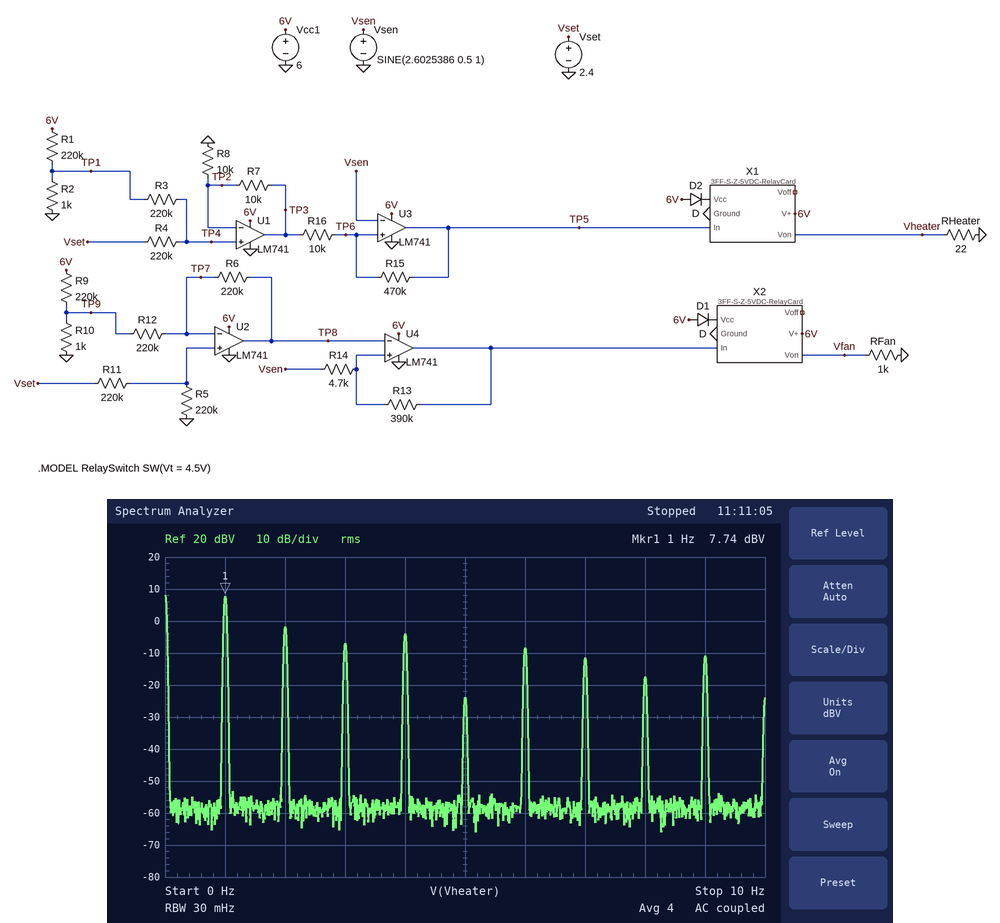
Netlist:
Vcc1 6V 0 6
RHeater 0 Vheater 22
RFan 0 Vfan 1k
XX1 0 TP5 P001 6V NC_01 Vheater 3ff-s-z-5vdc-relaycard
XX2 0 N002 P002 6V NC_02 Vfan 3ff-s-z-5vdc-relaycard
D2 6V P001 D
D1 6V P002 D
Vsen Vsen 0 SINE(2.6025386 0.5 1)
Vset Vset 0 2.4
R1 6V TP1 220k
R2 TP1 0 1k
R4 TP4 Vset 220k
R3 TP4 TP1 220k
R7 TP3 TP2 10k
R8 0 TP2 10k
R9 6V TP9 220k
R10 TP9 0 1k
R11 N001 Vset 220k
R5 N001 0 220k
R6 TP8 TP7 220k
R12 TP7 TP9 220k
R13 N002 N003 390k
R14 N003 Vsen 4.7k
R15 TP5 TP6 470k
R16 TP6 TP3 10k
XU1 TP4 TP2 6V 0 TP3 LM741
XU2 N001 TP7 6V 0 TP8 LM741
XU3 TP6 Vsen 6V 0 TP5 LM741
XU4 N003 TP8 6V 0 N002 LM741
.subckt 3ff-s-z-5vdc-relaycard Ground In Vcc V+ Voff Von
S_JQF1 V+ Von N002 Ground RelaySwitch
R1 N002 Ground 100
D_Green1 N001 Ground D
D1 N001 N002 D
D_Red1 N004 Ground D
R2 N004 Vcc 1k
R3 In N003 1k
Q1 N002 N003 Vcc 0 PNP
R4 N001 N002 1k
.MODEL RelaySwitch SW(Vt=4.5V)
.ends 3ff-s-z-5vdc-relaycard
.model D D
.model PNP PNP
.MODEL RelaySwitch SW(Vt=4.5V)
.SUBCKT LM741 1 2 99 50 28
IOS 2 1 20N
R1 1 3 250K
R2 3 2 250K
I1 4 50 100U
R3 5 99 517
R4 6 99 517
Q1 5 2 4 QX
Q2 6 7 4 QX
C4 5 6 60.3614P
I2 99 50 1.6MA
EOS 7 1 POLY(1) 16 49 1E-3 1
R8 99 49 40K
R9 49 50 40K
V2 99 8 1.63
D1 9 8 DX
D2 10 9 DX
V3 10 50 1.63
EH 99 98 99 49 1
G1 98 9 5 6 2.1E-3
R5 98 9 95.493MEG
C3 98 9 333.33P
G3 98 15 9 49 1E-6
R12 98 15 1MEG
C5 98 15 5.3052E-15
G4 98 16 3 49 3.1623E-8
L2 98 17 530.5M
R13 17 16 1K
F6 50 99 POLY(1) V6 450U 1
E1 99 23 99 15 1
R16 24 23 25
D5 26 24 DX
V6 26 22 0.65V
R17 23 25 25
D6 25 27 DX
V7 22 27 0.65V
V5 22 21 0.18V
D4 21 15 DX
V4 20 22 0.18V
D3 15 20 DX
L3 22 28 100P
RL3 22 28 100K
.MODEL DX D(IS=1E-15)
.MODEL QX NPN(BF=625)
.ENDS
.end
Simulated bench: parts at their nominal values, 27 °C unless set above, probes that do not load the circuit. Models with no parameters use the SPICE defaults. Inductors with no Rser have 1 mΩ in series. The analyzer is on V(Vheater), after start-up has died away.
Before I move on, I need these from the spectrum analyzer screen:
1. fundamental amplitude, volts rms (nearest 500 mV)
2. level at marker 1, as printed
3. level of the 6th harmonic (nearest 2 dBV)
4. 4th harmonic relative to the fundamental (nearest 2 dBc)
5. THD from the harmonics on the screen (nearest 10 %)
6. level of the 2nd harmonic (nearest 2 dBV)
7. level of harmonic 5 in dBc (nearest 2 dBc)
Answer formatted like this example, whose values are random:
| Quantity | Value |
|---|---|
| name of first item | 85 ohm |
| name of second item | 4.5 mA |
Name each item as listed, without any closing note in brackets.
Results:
| Quantity | Value |
|---|---|
| fundamental amplitude, volts rms | 2.5 V |
| level at marker 1, as printed | 7.74 dBV |
| level of the 6th harmonic | -8 dBV |
| 4th harmonic relative to the fundamental | -12 dBc |
| THD from the harmonics on the screen | 50 % |
| level of the 2nd harmonic | -2 dBV |
| level of harmonic 5 in dBc | -32 dBc |
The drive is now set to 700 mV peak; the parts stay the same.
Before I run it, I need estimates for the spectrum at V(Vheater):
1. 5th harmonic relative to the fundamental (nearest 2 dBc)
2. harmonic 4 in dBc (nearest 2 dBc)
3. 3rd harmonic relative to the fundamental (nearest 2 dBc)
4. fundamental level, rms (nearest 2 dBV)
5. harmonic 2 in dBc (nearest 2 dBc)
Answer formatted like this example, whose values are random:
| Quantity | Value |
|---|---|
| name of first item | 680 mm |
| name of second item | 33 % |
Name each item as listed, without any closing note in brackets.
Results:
| Quantity | Value |
|---|---|
| 5th harmonic relative to the fundamental | -22 dBc |
| harmonic 4 in dBc | -14 dBc |
| 3rd harmonic relative to the fundamental | -12 dBc |
| fundamental level, rms | 8 dBV |
| harmonic 2 in dBc | -12 dBc |
